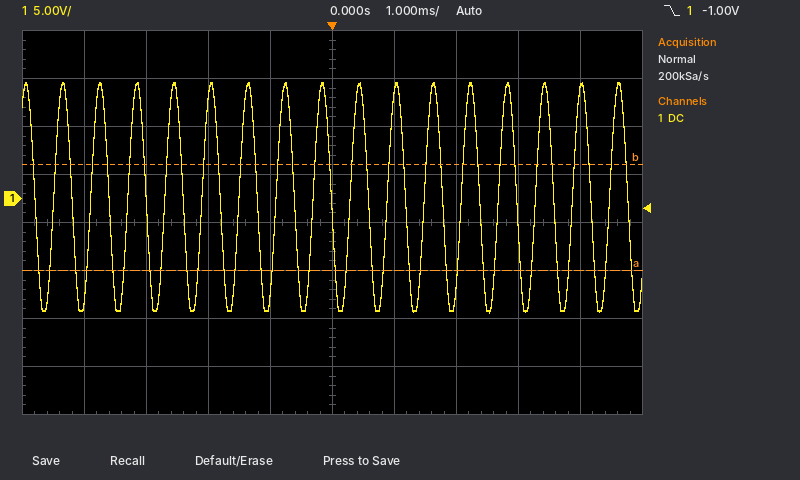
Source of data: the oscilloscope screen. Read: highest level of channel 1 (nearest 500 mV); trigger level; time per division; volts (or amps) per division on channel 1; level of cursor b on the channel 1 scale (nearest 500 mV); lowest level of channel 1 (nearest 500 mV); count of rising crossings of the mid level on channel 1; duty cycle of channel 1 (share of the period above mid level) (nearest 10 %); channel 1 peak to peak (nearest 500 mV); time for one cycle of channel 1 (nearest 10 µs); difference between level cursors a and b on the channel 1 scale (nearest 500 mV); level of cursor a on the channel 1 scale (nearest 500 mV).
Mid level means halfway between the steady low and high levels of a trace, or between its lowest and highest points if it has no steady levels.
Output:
12.0 V
-1.00 V
1 ms
5 V
3.5 V
-12.0 V
16
50 %
24.0 V
600 µs
11.0 V
-7.5 V
